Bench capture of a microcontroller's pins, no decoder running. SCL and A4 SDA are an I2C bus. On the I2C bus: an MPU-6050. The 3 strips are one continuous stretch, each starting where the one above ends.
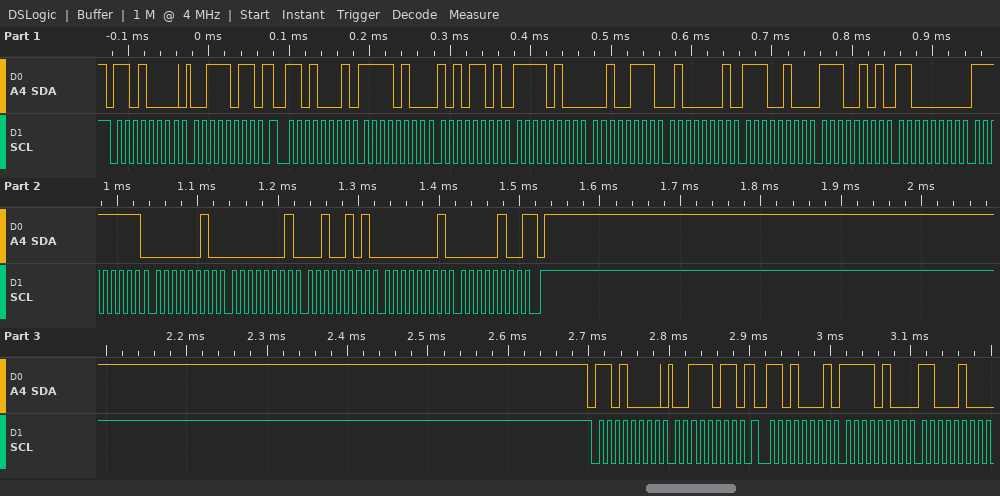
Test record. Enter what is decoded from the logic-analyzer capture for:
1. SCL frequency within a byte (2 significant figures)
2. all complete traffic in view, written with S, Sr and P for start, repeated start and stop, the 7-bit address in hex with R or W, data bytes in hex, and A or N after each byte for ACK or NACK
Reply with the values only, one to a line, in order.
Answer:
100 kHz
S 68W A 3B A Sr 68R A F4 A AD A F4 A 27 A 41 A E4 A E5 A C0 A FF A 02 A 01 A 25 A 01 A 04 N P S 68W A 3B A Sr 68R A F4 A C4 A
